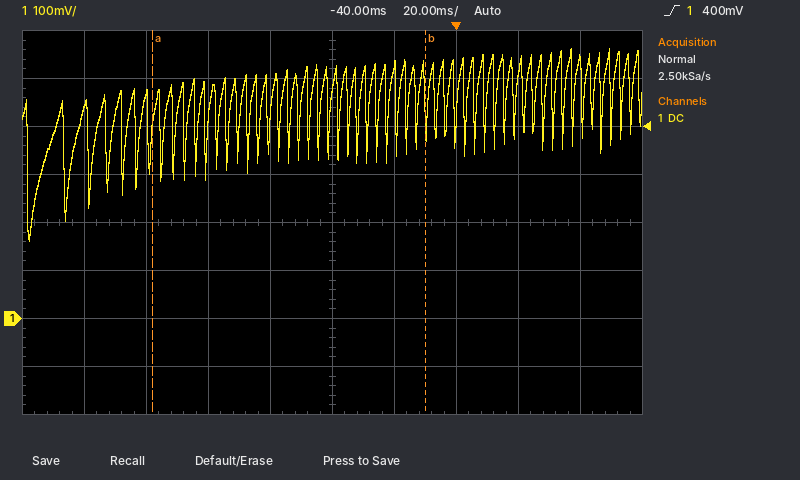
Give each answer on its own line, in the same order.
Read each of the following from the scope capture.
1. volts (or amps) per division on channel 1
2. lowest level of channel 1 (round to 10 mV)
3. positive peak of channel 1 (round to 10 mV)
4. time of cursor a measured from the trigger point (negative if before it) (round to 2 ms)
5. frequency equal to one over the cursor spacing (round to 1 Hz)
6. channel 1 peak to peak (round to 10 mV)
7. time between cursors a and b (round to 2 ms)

100 mV
160 mV
560 mV
-98 ms
11 Hz
400 mV
88 ms
